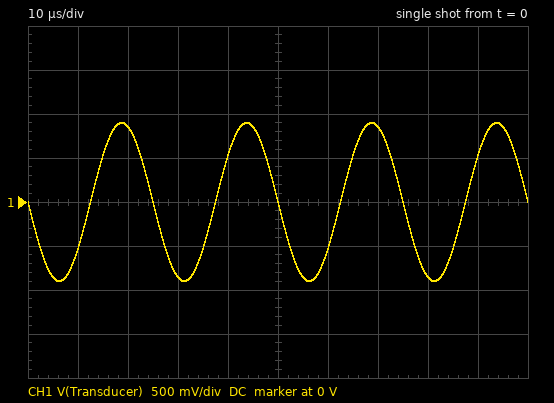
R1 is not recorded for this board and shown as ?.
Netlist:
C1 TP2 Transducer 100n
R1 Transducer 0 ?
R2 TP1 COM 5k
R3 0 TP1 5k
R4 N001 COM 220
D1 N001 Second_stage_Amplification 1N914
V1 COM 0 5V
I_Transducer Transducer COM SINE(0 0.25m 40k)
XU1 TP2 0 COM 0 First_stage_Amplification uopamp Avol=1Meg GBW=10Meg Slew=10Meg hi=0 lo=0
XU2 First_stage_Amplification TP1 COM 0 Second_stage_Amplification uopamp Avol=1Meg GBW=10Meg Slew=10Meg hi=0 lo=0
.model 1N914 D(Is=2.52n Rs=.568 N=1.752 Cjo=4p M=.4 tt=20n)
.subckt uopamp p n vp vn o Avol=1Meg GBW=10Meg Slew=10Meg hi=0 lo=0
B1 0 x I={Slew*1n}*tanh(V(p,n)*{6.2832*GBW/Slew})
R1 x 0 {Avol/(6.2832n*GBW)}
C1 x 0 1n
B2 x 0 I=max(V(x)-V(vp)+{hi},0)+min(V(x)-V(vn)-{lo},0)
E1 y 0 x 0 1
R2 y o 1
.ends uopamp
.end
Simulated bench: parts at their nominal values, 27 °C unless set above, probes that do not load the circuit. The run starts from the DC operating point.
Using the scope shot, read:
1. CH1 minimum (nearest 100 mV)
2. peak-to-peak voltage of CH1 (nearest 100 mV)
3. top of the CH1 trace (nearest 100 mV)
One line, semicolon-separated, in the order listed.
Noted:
-900 mV; 1.8 V; 900 mV
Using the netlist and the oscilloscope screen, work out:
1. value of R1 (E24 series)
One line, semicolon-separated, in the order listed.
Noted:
3.6 kΩ
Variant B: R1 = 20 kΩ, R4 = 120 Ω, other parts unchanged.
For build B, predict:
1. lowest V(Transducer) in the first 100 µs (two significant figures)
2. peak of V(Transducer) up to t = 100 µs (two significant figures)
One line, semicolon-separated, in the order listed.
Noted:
-5.0 V; 5.0 V
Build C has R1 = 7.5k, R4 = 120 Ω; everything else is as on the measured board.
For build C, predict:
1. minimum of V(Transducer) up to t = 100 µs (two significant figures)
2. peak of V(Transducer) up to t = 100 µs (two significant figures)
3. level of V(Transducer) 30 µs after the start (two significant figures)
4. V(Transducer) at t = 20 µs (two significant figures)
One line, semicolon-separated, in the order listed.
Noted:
-1.9 V; 1.9 V; -1.8 V; 1.8 V
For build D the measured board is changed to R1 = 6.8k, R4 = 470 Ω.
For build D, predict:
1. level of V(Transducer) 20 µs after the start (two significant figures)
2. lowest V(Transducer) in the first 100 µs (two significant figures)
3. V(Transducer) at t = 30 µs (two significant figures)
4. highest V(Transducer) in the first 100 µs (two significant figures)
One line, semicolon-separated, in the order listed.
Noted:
1.6 V; -1.7 V; -1.6 V; 1.7 V
